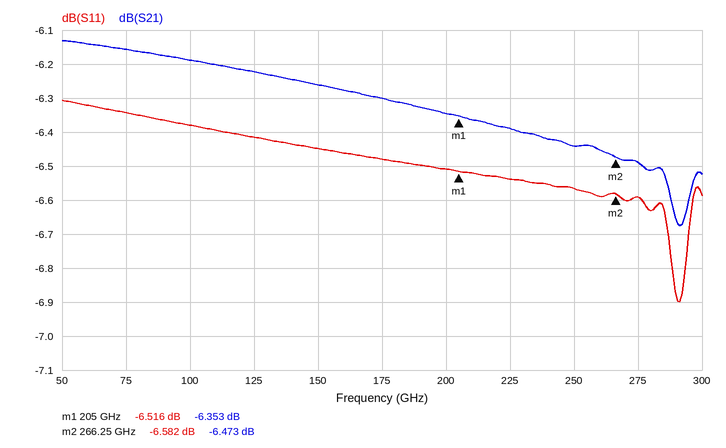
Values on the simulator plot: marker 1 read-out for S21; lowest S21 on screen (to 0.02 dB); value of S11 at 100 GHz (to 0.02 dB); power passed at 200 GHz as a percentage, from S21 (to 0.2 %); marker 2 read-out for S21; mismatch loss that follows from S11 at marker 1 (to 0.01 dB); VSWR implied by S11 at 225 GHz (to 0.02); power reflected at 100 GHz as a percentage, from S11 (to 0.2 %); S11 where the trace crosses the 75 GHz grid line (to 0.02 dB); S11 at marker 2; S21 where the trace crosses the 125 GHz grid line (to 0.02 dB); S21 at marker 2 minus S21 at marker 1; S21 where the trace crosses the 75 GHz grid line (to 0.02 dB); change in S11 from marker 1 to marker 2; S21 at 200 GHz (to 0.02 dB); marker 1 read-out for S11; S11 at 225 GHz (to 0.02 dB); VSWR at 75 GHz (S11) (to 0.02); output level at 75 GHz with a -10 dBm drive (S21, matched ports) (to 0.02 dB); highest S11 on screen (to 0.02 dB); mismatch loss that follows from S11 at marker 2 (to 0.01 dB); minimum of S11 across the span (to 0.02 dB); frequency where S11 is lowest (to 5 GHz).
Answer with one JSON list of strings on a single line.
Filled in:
["-6.353 dB", "-6.68 dB", "-6.38 dB", "23.2 %", "-6.473 dB", "1.10 dB", "2.78", "23.0 %", "-6.34 dB", "-6.582 dB", "-6.22 dB", "-0.120 dB", "-6.16 dB", "-0.066 dB", "-6.34 dB", "-6.516 dB", "-6.54 dB", "2.86", "-16.16 dBm", "-6.30 dB", "1.08 dB", "-6.90 dB", "290 GHz"]
